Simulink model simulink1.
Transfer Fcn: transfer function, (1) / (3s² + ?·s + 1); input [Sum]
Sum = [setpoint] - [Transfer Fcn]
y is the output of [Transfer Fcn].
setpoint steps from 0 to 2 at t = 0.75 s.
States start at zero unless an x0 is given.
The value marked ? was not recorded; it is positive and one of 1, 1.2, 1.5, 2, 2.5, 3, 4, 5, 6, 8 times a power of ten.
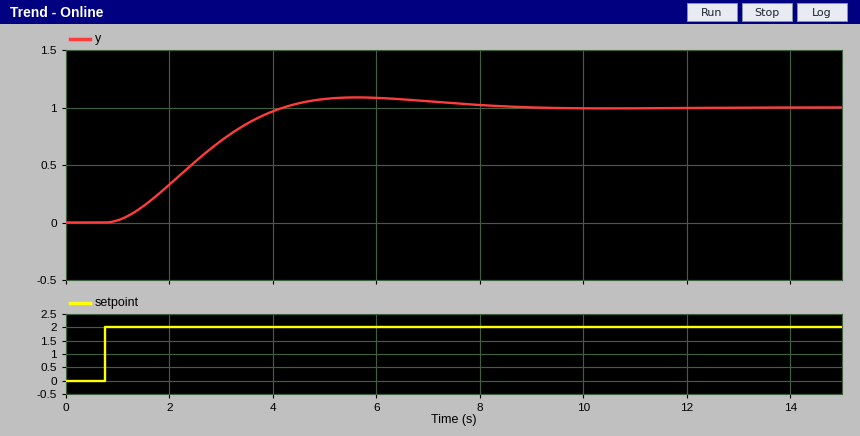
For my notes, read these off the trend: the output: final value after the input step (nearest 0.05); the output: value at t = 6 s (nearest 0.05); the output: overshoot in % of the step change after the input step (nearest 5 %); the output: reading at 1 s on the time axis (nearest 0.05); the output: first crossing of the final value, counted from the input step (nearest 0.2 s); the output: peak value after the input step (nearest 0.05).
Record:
1.00
1.10
10 %
0.00
3.4 s
1.10
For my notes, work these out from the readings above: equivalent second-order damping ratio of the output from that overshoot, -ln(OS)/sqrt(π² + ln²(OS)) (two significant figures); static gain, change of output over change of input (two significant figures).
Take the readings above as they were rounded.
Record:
0.59
0.50
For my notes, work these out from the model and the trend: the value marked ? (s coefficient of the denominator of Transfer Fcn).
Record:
3
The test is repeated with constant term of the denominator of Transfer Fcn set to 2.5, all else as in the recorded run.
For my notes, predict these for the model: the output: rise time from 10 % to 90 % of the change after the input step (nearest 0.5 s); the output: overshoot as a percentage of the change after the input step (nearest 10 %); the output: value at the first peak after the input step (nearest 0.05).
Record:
1.5 s
20 %
0.70
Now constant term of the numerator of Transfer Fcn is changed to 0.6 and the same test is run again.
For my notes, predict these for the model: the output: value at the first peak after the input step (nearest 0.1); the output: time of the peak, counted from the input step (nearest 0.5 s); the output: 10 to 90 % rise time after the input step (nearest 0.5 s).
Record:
0.8
6.0 s
3.0 s
